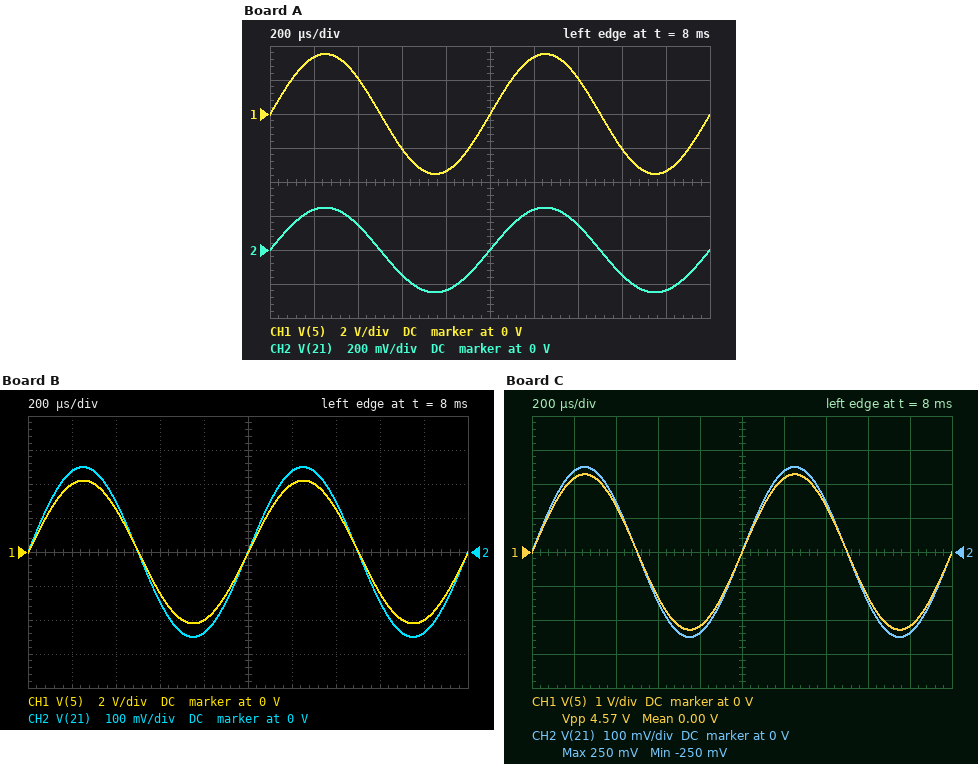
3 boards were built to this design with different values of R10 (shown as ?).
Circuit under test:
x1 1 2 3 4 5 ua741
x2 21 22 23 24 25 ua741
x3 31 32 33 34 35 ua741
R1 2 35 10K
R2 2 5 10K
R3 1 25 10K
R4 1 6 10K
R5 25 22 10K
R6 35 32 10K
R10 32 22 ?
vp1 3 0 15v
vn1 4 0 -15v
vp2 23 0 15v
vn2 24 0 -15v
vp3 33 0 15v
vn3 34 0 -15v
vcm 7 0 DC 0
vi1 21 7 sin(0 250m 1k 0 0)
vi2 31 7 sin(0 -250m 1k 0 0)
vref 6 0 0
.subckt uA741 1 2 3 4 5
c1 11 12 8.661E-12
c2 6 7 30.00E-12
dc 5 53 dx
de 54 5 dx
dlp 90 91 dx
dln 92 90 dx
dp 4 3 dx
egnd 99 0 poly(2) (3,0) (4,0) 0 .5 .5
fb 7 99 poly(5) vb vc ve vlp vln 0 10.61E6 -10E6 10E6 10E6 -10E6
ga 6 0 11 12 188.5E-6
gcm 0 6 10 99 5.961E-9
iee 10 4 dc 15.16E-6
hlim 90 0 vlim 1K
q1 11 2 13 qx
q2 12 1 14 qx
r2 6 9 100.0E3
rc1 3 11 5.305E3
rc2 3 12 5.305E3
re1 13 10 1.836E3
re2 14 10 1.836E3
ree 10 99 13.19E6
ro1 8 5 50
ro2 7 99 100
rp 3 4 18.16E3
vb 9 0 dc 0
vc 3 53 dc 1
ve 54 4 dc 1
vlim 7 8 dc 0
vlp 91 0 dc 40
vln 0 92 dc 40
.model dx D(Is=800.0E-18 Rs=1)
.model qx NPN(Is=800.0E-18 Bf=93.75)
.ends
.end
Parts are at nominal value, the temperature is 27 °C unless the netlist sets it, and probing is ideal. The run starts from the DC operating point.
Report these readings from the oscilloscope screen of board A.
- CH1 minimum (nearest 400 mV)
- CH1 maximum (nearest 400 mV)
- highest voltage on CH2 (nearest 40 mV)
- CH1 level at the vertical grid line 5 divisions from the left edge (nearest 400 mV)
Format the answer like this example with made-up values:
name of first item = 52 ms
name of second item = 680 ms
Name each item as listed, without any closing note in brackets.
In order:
CH1 minimum = -3.6 V
CH1 maximum = 3.6 V
highest voltage on CH2 = 240 mV
CH1 level at the vertical grid line 5 divisions from the left edge = 0 V
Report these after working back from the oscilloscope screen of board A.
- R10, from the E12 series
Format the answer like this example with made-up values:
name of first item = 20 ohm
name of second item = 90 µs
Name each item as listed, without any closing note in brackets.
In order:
R10, from the E12 series = 3.3 kΩ
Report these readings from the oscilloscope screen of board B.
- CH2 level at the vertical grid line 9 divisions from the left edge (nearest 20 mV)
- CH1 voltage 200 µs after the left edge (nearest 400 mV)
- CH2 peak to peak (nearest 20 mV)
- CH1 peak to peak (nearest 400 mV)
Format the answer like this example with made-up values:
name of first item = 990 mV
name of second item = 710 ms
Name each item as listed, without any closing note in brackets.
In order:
CH2 level at the vertical grid line 9 divisions from the left edge = -240 mV
CH1 voltage 200 µs after the left edge = 4.0 V
CH2 peak to peak = 500 mV
CH1 peak to peak = 8.4 V
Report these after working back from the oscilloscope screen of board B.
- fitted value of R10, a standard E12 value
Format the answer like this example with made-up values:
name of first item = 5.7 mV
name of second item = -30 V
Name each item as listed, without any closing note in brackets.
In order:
fitted value of R10, a standard E12 value = 2.7 kΩ
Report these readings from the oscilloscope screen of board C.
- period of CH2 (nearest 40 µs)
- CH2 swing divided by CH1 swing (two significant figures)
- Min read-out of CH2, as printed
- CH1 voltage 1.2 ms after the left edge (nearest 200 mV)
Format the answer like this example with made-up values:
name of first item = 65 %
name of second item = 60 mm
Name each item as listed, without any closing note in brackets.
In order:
period of CH2 = 1.00 ms
CH2 swing divided by CH1 swing = 0.11
Min read-out of CH2, as printed = -250 mV
CH1 voltage 1.2 ms after the left edge = 2.2 V
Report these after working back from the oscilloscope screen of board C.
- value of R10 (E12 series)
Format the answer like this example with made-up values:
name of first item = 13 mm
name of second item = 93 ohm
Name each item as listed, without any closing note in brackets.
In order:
value of R10 = 5.6 kΩ
